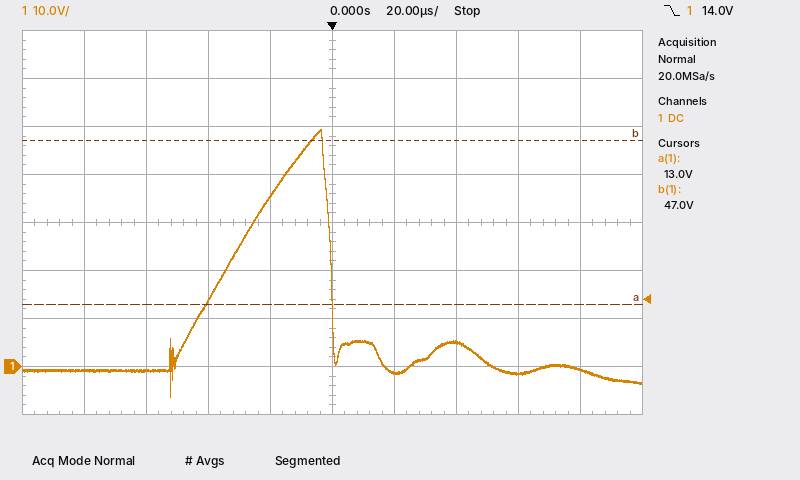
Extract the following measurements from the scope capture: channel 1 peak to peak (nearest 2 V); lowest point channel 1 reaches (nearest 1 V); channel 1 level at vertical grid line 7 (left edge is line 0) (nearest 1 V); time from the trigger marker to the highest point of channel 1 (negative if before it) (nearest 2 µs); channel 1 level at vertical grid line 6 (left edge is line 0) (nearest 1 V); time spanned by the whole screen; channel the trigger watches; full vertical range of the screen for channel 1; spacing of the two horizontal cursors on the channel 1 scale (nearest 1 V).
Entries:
56 V
-6 V
5 V
-4 µs
-1 V
200 µs
channel 1
80 V
34 V
